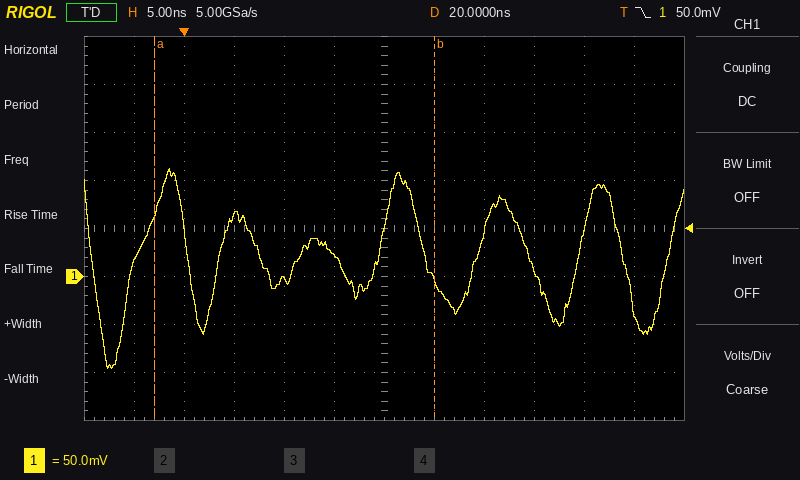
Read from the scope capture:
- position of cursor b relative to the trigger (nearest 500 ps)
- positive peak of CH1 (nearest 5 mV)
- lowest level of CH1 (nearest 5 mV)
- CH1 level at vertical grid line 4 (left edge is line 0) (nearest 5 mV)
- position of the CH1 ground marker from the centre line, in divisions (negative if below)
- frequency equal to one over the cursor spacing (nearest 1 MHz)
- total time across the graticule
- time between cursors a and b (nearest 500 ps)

+25.0 ns
110 mV
-95 mV
-5 mV
-1.0 div
36 MHz
60 ns
28.0 ns
